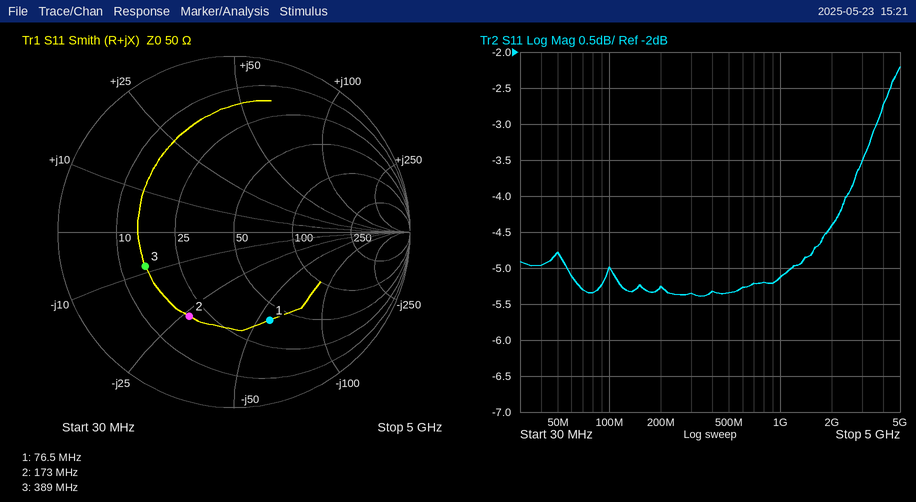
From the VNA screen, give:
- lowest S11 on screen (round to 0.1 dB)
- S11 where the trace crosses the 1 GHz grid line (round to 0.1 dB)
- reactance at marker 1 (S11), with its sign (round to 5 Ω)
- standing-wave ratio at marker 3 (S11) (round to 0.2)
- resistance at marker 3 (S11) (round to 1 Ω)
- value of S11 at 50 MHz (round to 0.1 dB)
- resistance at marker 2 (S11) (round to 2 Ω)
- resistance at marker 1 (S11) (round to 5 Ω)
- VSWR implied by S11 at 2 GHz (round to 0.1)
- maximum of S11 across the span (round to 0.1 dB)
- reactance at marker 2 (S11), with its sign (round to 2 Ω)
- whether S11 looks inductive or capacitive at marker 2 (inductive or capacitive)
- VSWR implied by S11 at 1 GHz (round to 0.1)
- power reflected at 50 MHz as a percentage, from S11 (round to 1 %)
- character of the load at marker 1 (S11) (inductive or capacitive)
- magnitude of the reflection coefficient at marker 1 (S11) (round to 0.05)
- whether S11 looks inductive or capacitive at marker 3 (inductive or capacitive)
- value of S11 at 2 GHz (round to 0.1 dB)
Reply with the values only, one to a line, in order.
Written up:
-5.4 dB
-5.1 dB
-55 Ω
3.4
15 Ω
-4.8 dB
20 Ω
40 Ω
4.0
-2.2 dB
-26 Ω
capacitive
3.5
33 %
capacitive
0.55
capacitive
-4.4 dB
